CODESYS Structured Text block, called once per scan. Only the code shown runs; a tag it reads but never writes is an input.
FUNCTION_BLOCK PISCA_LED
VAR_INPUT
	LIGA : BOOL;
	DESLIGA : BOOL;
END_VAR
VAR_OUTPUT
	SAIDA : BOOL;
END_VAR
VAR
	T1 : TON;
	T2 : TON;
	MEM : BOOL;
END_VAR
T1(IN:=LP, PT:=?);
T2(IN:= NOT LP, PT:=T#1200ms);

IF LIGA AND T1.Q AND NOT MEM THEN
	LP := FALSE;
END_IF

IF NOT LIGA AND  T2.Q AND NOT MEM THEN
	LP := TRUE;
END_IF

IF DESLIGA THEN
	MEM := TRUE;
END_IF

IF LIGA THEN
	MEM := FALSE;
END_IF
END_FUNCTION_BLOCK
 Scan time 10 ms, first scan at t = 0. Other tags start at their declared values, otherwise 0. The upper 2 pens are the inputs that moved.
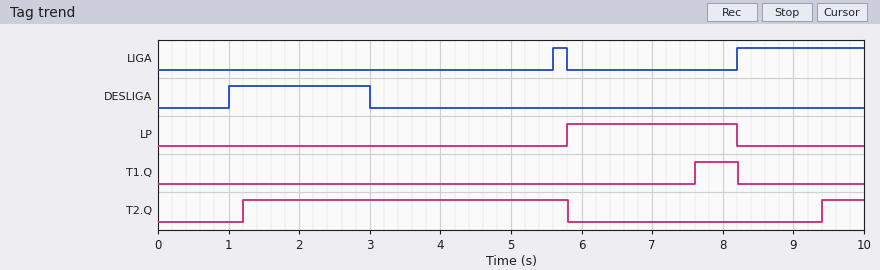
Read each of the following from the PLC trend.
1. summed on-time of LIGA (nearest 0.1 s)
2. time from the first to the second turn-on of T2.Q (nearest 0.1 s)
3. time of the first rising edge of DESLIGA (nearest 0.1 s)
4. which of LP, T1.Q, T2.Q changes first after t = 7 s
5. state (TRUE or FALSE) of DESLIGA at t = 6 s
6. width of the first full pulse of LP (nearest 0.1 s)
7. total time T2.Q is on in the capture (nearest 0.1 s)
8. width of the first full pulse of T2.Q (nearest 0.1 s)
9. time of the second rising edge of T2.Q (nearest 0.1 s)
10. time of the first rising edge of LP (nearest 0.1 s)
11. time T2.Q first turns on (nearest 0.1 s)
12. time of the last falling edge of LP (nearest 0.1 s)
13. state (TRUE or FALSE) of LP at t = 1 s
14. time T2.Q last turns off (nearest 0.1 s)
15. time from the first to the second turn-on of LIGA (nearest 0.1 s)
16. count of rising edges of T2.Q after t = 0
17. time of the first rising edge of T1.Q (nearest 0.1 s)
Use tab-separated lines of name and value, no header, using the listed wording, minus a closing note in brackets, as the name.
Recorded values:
summed on-time of LIGA	2.0 s
time from the first to the second turn-on of T2.Q	8.2 s
time of the first rising edge of DESLIGA	1.0 s
which of LP, T1.Q, T2.Q changes first after t = 7 s	T1.Q
state (TRUE or FALSE) of DESLIGA at t = 6 s	FALSE
width of the first full pulse of LP	2.4 s
total time T2.Q is on in the capture	5.2 s
width of the first full pulse of T2.Q	4.6 s
time of the second rising edge of T2.Q	9.4 s
time of the first rising edge of LP	5.8 s
time T2.Q first turns on	1.2 s
time of the last falling edge of LP	8.2 s
state (TRUE or FALSE) of LP at t = 1 s	FALSE
time T2.Q last turns off	5.8 s
time from the first to the second turn-on of LIGA	2.6 s
count of rising edges of T2.Q after t = 0	2
time of the first rising edge of T1.Q	7.6 s
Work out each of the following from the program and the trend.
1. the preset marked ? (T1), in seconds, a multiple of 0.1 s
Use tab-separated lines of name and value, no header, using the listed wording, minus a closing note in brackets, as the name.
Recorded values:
the preset marked ? (T1), in seconds, a multiple of 0.1 s	1.8 s
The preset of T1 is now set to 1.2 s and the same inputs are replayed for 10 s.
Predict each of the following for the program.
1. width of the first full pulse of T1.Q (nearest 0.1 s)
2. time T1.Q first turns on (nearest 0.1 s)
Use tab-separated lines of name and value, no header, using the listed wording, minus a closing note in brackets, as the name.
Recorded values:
width of the first full pulse of T1.Q	1.2 s
time T1.Q first turns on	7.0 s
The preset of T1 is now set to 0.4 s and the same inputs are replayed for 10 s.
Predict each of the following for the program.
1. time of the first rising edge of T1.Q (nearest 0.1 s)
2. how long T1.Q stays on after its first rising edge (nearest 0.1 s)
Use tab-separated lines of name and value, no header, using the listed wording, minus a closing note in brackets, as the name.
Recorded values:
time of the first rising edge of T1.Q	6.2 s
how long T1.Q stays on after its first rising edge	2.0 s
